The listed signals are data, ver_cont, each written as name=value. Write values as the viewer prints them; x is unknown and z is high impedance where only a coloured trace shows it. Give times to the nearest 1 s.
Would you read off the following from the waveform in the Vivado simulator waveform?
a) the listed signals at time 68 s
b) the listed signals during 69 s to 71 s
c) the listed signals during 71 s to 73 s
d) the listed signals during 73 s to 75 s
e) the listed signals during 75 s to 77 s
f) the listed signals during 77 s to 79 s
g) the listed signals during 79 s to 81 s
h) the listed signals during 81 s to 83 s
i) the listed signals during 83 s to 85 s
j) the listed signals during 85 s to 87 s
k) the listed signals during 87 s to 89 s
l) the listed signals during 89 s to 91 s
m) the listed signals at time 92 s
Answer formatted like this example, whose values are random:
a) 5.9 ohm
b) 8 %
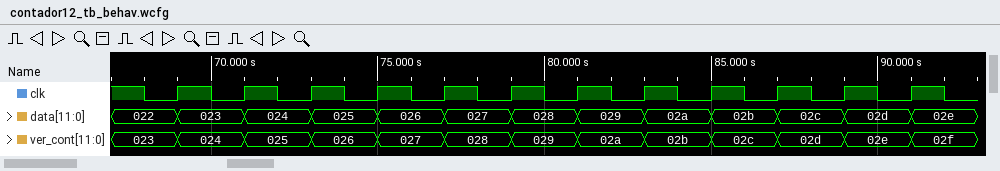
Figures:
a) data=022, ver_cont=023
b) data=023, ver_cont=024
c) data=024, ver_cont=025
d) data=025, ver_cont=026
e) data=026, ver_cont=027
f) data=027, ver_cont=028
g) data=028, ver_cont=029
h) data=029, ver_cont=02a
i) data=02a, ver_cont=02b
j) data=02b, ver_cont=02c
k) data=02c, ver_cont=02d
l) data=02d, ver_cont=02e
m) data=02e, ver_cont=02f
